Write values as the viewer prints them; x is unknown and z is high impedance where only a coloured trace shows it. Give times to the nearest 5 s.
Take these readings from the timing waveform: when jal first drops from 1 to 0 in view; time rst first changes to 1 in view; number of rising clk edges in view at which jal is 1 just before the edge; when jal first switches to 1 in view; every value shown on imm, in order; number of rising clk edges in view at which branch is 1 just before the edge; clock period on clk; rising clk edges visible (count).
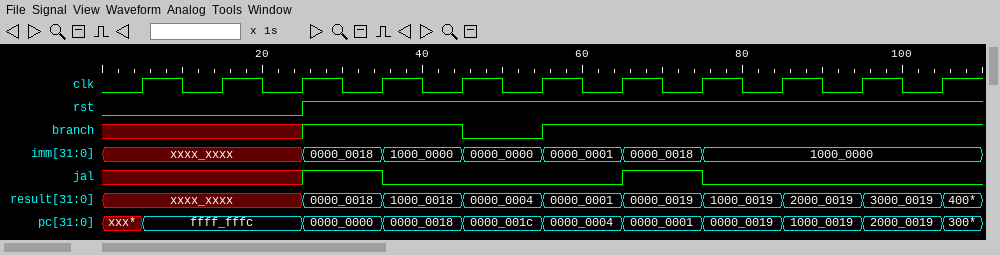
35 s
25 s
2
25 s
xxxx_xxxx, 0000_0018, 1000_0000, 0000_0000, 0000_0001, 0000_0018, 1000_0000
7
10 s
11
